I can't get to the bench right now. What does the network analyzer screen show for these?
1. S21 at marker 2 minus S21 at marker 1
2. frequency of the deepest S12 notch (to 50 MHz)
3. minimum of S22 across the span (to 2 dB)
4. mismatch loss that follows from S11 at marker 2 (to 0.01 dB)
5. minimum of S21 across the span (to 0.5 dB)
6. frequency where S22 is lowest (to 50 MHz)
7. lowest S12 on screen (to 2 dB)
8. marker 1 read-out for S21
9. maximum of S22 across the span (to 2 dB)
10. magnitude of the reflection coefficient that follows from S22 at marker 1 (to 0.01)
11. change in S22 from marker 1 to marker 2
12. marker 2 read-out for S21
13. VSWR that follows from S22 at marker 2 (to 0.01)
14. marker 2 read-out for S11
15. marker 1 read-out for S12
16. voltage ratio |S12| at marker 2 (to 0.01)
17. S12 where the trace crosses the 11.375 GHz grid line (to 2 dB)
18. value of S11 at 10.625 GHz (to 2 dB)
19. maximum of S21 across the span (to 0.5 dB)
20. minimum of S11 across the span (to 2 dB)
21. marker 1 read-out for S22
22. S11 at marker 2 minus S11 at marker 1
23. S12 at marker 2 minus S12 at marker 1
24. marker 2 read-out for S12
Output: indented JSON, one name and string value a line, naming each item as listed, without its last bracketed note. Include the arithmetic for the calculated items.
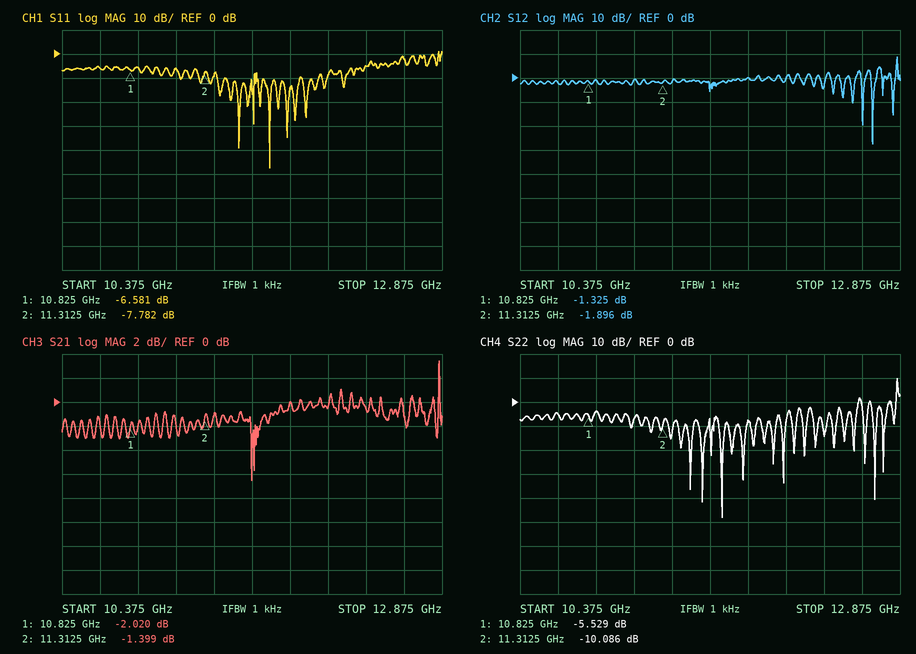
{
  "S21 at marker 2 minus S21 at marker 1": "-1.399 − (-2.02) = 0.621 dB",
  "frequency of the deepest S12 notch": "12.70 GHz",
  "minimum of S22 across the span": "-48 dB",
  "mismatch loss that follows from S11 at marker 2": "−10 log10(1 − 10^(-7.782/10)) ≈ 0.79 dB",
  "minimum of S21 across the span": "-6.5 dB",
  "frequency where S22 is lowest": "11.70 GHz",
  "lowest S12 on screen": "-28 dB",
  "marker 1 read-out for S21": "-2.020 dB",
  "maximum of S22 across the span": "10 dB",
  "magnitude of the reflection coefficient that follows from S22 at marker 1": "10^(-5.529/20) ≈ 0.53",
  "change in S22 from marker 1 to marker 2": "-10.086 − (-5.529) = -4.557 dB",
  "marker 2 read-out for S21": "-1.399 dB",
  "VSWR that follows from S22 at marker 2": "(1 + 0.3131)/(1 − 0.3131) ≈ 1.91",
  "marker 2 read-out for S11": "-7.782 dB",
  "marker 1 read-out for S12": "-1.325 dB",
  "voltage ratio |S12| at marker 2": "10^(-1.896/20) ≈ 0.80",
  "S12 where the trace crosses the 11.375 GHz grid line": "-2 dB",
  "value of S11 at 10.625 GHz": "-6 dB",
  "maximum of S21 across the span": "3.5 dB",
  "minimum of S11 across the span": "-48 dB",
  "marker 1 read-out for S22": "-5.529 dB",
  "S11 at marker 2 minus S11 at marker 1": "-7.782 − (-6.581) = -1.201 dB",
  "S12 at marker 2 minus S12 at marker 1": "-1.896 − (-1.325) = -0.571 dB",
  "marker 2 read-out for S12": "-1.896 dB"
}
